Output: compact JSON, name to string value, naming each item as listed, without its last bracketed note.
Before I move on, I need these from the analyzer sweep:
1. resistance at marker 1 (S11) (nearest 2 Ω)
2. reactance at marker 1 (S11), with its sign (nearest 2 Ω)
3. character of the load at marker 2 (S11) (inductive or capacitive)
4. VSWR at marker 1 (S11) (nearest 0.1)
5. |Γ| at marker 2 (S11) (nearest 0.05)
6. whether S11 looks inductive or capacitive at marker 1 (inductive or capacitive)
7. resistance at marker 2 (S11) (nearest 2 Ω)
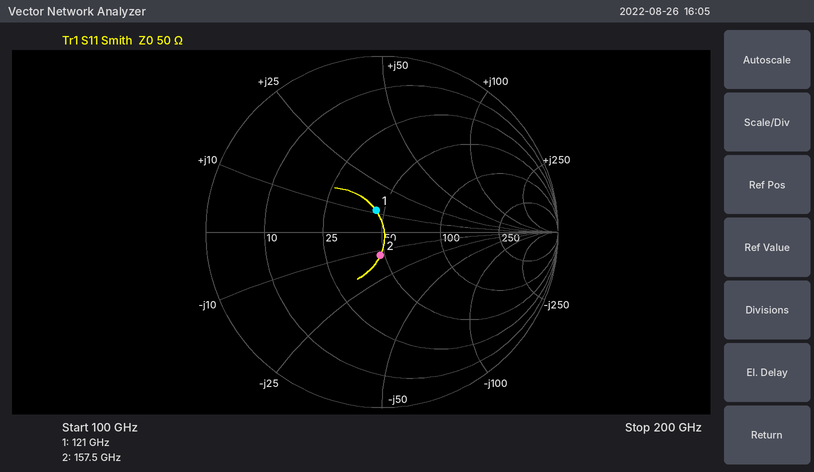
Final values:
{"resistance at marker 1 (S11)": "46 Ω", "reactance at marker 1 (S11), with its sign": "+12 Ω", "character of the load at marker 2 (S11)": "capacitive", "VSWR at marker 1 (S11)": "1.3", "|Γ| at marker 2 (S11)": "0.15", "whether S11 looks inductive or capacitive at marker 1": "inductive", "resistance at marker 2 (S11)": "48 Ω"}
